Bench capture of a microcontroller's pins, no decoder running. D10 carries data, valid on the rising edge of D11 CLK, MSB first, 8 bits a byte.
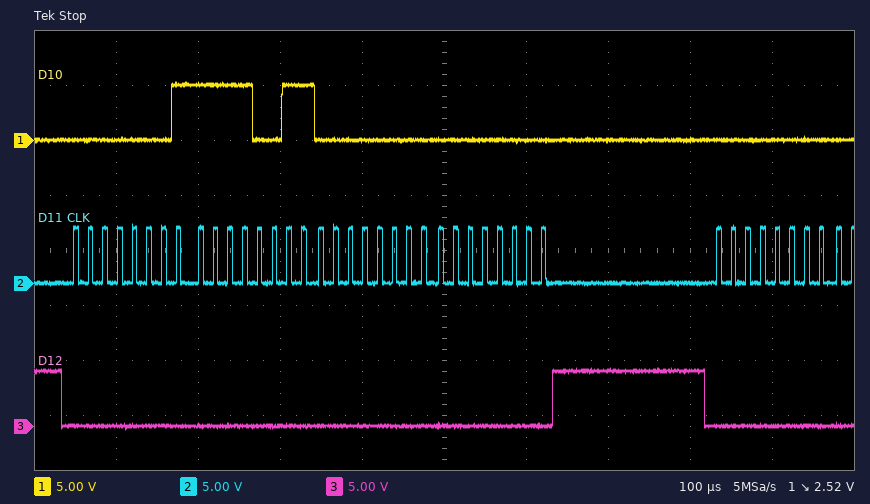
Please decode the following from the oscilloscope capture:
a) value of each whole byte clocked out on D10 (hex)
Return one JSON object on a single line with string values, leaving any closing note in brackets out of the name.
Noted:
{"value of each whole byte clocked out on D10": "01 F3 00 00 00"}
